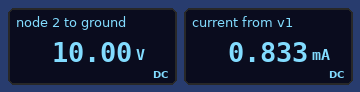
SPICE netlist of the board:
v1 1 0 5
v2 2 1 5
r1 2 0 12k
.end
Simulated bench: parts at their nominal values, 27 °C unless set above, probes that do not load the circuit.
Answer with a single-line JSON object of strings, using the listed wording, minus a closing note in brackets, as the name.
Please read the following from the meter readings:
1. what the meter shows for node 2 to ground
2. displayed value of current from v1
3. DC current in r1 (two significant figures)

{"what the meter shows for node 2 to ground": "10.00 V", "displayed value of current from v1": "0.833 mA", "DC current in r1": "830 µA"}
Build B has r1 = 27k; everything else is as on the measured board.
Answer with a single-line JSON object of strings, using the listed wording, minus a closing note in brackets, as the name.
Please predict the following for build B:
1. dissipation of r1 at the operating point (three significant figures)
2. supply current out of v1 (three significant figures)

{"dissipation of r1 at the operating point": "3.70 mW", "supply current out of v1": "370 µA"}
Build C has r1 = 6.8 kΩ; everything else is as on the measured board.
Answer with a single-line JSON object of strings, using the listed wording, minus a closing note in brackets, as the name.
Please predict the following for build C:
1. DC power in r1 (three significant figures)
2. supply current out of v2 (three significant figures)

{"DC power in r1": "14.7 mW", "supply current out of v2": "1.47 mA"}
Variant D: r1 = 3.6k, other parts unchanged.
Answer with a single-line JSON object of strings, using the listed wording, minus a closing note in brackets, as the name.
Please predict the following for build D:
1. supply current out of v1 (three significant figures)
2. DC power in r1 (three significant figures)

{"supply current out of v1": "2.78 mA", "DC power in r1": "27.8 mW"}
